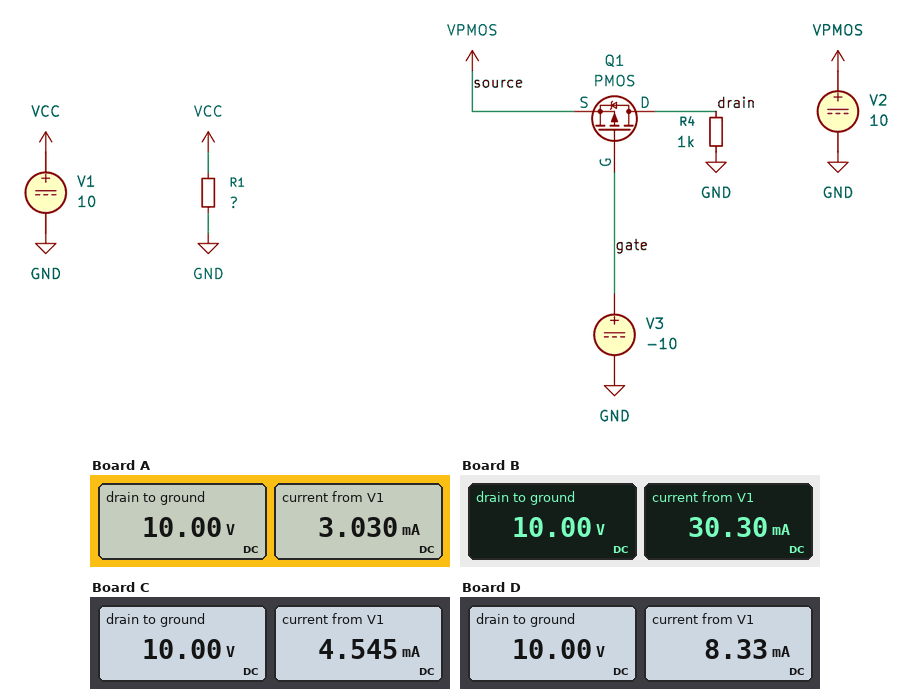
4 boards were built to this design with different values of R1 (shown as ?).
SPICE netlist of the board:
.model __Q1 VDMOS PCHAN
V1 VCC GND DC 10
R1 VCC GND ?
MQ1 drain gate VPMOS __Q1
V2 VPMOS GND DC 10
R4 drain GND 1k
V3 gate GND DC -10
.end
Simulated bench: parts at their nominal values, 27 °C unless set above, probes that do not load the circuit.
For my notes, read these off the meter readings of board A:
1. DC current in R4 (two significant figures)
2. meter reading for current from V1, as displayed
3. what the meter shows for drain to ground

10 mA
3.030 mA
10.00 V
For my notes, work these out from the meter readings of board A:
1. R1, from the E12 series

3.3 kΩ
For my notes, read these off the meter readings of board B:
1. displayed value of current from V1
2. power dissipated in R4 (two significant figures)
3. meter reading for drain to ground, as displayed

30.30 mA
100 mW
10.00 V
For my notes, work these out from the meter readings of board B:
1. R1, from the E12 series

330 Ω
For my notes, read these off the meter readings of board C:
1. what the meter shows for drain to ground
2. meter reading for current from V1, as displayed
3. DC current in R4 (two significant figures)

10.00 V
4.545 mA
10 mA
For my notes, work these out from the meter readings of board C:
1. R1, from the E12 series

2.2 kΩ
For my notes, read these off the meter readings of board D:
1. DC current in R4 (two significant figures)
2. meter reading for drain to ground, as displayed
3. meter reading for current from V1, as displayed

10 mA
10.00 V
8.33 mA
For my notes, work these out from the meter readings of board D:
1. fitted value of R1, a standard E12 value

1.2 kΩ
